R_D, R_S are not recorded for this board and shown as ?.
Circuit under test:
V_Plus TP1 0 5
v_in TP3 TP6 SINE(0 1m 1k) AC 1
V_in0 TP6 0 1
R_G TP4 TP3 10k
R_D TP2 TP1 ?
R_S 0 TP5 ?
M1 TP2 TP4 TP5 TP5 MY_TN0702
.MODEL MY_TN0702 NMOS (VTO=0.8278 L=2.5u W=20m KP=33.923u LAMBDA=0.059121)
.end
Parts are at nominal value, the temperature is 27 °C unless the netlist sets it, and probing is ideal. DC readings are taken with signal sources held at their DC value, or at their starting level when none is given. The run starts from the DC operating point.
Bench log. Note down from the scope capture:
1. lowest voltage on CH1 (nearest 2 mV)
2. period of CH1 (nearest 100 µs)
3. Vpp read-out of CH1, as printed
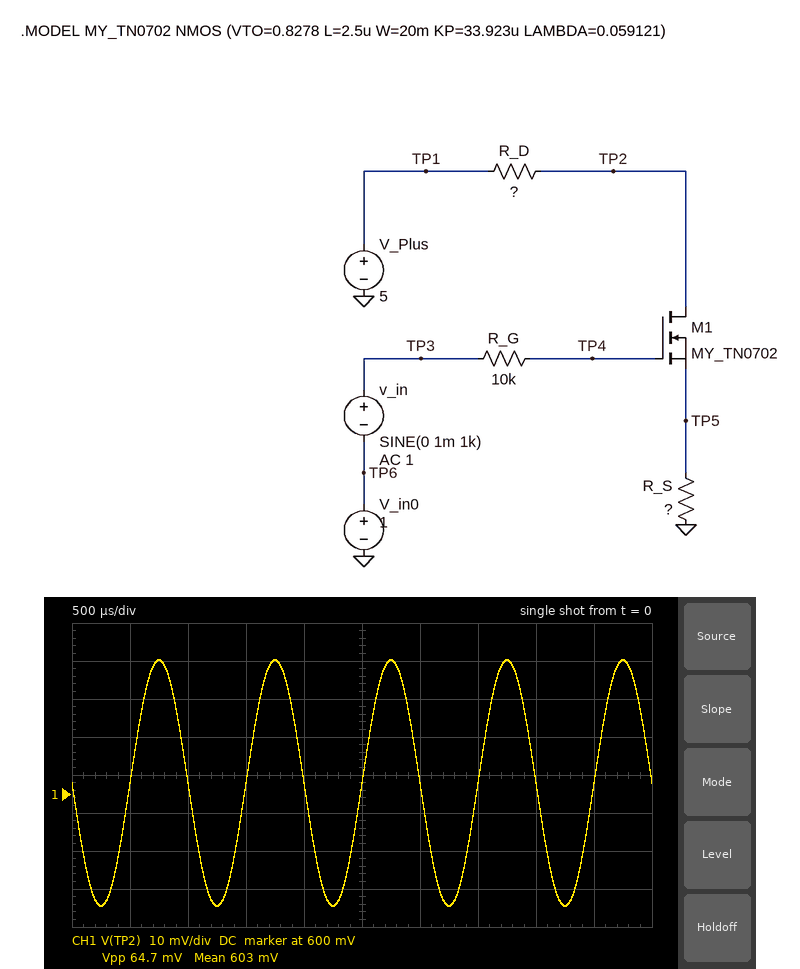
570 mV
1.0 ms
64.7 mV
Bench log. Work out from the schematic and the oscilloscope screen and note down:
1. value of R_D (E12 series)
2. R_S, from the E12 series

3.3 kΩ
56 Ω
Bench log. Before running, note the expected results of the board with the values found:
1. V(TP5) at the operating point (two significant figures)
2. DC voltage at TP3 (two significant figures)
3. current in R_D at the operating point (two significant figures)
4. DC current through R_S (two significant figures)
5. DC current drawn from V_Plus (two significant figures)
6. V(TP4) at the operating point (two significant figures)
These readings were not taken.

75 mV
1.0 V
1.3 mA
1.3 mA
1.3 mA
1.0 V
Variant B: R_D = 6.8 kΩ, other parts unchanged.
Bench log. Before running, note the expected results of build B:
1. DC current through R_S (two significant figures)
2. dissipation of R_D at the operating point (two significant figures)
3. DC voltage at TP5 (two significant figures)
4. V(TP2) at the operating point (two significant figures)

730 µA
3.6 mW
41 mV
63 mV
